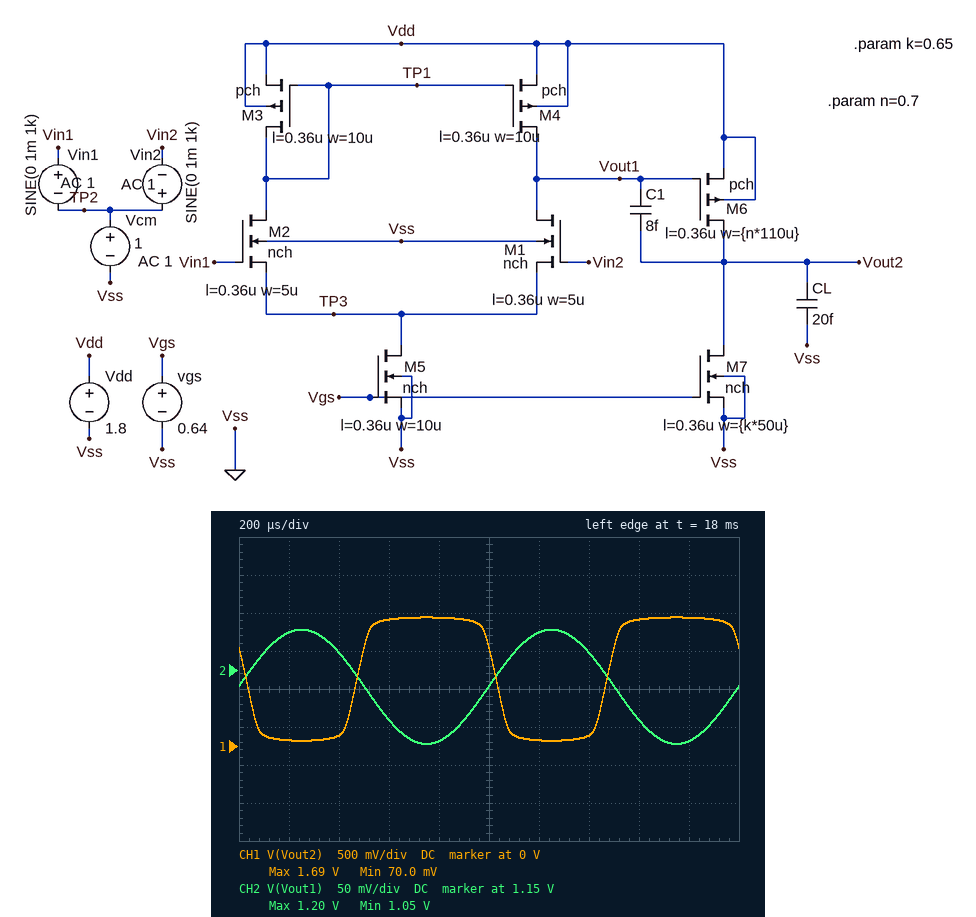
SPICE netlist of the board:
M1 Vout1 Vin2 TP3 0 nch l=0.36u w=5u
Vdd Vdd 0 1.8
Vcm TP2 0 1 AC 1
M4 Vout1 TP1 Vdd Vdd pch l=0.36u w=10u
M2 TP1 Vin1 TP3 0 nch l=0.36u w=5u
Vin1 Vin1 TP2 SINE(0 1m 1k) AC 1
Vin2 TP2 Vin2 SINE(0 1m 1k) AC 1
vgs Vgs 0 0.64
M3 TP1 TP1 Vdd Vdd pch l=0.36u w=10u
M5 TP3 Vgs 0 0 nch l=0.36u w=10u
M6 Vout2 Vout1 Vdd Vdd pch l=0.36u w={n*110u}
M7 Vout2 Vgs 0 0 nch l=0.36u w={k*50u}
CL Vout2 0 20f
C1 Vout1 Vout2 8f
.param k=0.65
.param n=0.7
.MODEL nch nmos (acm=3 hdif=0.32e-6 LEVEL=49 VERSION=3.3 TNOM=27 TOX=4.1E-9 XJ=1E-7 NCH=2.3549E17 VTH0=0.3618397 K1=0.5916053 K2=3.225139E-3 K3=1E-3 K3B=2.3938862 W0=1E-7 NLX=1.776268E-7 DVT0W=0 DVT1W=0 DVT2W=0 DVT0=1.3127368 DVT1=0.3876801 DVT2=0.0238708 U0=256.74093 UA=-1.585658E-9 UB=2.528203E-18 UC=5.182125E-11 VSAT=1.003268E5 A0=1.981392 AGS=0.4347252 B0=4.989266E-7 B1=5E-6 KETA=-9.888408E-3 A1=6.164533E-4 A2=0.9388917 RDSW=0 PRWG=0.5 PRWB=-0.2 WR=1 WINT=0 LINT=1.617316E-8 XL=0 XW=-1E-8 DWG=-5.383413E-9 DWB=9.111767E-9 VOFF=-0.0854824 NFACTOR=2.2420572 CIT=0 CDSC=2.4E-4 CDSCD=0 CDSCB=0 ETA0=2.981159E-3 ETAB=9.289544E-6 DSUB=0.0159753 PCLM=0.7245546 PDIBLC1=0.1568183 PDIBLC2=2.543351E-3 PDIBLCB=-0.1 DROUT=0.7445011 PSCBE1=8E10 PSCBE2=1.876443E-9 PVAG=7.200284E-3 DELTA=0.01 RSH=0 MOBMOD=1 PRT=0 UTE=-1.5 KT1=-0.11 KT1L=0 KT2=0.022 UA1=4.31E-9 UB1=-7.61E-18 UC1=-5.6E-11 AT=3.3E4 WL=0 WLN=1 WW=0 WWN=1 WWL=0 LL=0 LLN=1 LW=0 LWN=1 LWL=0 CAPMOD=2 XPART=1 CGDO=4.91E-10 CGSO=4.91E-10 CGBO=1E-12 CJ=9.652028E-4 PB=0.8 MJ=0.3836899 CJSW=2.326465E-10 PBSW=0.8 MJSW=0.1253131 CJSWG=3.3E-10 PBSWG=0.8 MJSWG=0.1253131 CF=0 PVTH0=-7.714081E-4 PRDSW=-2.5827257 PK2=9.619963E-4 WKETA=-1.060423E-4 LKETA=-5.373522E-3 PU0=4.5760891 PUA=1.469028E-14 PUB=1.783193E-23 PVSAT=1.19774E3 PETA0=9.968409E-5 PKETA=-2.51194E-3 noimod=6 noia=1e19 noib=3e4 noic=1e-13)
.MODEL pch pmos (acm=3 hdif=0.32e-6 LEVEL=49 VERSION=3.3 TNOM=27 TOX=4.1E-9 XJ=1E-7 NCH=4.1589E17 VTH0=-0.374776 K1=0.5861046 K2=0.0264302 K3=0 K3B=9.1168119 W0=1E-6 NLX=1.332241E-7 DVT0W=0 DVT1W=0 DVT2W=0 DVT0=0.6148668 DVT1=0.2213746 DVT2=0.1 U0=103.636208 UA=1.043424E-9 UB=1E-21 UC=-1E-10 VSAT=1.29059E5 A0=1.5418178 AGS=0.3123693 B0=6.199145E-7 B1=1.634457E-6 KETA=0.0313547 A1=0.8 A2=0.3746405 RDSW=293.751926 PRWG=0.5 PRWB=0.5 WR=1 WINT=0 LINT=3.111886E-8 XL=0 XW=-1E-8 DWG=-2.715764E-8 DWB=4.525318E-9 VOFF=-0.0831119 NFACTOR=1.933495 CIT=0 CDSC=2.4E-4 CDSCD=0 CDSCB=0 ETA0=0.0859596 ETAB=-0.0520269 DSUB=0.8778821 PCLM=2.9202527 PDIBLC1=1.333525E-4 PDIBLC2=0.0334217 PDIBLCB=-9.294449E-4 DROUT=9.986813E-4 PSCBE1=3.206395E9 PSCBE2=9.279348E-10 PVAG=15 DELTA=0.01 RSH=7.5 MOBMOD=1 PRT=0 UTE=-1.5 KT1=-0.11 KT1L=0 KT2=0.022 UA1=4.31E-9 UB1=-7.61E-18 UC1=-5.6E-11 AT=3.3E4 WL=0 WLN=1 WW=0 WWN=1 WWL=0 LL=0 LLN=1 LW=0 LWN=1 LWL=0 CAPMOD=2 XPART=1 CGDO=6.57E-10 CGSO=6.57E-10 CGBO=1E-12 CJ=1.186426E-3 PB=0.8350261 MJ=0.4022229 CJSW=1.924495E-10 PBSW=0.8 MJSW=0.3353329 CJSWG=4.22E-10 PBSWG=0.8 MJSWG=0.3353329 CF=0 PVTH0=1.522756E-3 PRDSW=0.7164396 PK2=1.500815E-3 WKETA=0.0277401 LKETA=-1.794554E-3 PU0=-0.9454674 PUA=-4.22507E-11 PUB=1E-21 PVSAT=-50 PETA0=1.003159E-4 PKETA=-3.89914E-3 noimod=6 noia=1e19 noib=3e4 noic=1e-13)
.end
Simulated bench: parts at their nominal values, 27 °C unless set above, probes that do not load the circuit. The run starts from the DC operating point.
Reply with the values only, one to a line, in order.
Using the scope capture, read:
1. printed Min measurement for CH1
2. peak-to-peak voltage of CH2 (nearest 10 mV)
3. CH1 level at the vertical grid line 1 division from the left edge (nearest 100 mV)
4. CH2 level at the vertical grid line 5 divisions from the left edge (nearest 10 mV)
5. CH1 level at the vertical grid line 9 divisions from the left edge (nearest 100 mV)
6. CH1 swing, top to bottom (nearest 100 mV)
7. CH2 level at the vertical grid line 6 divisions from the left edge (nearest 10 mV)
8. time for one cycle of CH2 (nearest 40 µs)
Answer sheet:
70.0 mV
150 mV
100 mV
1.13 V
1.7 V
1.6 V
1.20 V
1.00 ms
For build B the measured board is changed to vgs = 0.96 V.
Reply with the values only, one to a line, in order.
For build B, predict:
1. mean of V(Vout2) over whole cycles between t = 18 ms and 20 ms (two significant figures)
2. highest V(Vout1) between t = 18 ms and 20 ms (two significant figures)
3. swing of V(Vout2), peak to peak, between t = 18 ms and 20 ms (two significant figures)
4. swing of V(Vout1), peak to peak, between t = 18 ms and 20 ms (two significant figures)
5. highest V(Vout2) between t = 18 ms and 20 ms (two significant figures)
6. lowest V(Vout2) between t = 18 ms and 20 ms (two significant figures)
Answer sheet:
200 mV
910 mV
130 mV
110 mV
270 mV
140 mV
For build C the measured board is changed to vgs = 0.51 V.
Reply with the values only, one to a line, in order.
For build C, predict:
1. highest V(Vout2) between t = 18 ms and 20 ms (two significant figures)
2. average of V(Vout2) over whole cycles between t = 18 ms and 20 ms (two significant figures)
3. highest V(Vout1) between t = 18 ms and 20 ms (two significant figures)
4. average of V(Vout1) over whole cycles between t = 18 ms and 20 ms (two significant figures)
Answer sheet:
1.8 V
940 mV
1.4 V
1.3 V
